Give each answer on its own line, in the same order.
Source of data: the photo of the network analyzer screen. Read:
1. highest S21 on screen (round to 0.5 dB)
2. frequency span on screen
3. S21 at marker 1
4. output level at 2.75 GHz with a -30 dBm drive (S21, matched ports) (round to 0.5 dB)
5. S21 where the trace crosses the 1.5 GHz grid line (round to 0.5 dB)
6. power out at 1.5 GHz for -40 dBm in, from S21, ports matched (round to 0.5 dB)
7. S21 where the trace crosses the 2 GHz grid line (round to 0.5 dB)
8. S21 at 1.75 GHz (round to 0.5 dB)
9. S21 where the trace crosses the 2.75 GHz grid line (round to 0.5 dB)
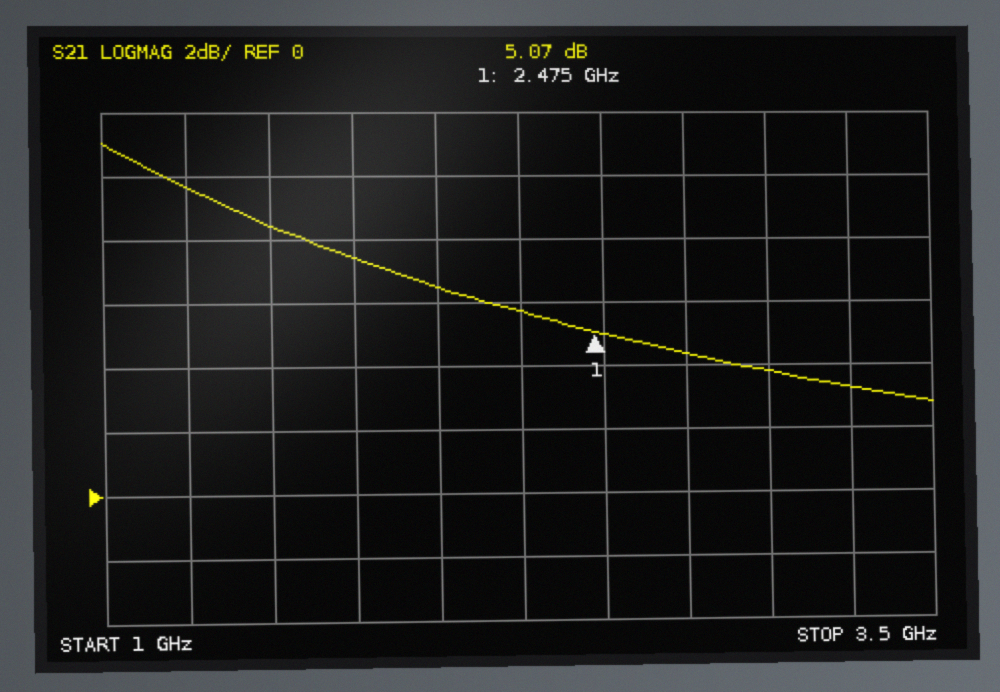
11.0 dB
2.5 GHz
5.07 dB
-25.5 dBm
8.5 dB
-31.5 dBm
6.5 dB
7.5 dB
4.5 dB
